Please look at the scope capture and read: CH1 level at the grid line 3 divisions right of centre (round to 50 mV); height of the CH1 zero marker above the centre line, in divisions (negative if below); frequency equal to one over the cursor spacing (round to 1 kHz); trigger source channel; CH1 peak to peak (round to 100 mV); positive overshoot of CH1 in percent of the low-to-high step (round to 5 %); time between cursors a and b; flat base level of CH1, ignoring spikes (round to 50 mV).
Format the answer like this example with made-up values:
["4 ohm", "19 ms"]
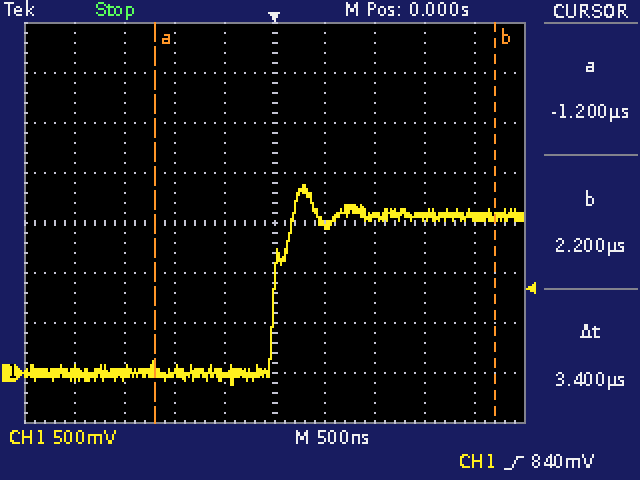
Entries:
["1.55 V", "-3.0 div", "294 kHz", "CH1", "2.00 V", "20 %", "3.4 µs", "0 mV"]
